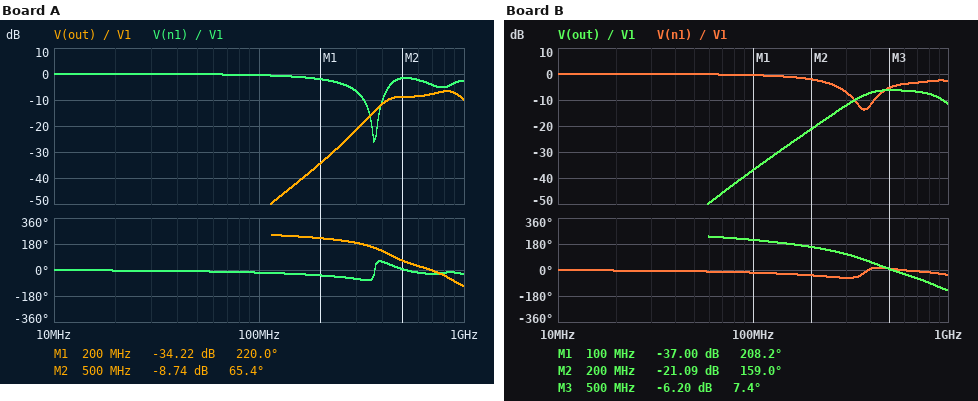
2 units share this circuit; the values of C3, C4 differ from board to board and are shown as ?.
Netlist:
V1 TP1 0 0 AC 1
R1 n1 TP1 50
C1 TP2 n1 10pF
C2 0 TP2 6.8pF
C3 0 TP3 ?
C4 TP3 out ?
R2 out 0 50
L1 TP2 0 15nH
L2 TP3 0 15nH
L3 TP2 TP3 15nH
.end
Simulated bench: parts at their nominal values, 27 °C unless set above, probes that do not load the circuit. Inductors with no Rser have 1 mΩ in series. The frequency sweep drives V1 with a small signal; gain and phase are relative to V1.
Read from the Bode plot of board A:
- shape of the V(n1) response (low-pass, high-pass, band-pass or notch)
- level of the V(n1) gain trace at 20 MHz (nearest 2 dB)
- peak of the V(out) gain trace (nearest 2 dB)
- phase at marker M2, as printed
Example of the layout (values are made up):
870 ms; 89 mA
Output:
notch; 0 dB; -6 dB; 65.4 deg
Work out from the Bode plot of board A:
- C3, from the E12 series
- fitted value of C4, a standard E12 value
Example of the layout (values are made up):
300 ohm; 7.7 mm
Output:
3.3 pF; 3.3 pF
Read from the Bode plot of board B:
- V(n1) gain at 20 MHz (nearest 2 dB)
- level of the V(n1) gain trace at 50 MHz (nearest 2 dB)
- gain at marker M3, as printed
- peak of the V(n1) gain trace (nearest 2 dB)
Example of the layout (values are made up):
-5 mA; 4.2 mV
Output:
0 dB; 0 dB; -6.20 dB; 0 dB
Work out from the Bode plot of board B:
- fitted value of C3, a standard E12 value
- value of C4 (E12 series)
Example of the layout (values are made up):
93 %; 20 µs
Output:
4.7 pF; 27 pF
